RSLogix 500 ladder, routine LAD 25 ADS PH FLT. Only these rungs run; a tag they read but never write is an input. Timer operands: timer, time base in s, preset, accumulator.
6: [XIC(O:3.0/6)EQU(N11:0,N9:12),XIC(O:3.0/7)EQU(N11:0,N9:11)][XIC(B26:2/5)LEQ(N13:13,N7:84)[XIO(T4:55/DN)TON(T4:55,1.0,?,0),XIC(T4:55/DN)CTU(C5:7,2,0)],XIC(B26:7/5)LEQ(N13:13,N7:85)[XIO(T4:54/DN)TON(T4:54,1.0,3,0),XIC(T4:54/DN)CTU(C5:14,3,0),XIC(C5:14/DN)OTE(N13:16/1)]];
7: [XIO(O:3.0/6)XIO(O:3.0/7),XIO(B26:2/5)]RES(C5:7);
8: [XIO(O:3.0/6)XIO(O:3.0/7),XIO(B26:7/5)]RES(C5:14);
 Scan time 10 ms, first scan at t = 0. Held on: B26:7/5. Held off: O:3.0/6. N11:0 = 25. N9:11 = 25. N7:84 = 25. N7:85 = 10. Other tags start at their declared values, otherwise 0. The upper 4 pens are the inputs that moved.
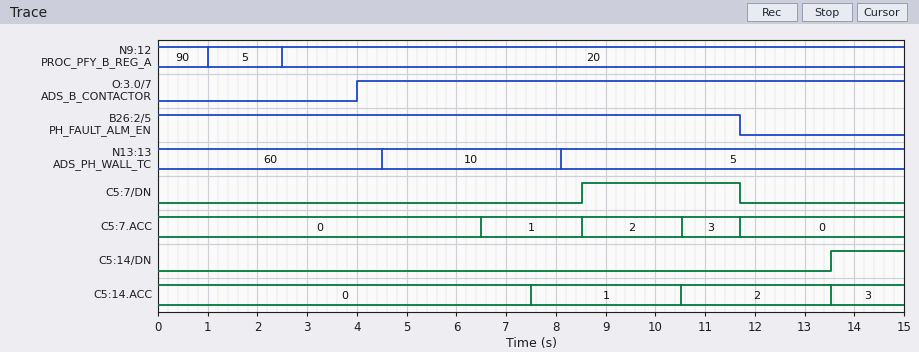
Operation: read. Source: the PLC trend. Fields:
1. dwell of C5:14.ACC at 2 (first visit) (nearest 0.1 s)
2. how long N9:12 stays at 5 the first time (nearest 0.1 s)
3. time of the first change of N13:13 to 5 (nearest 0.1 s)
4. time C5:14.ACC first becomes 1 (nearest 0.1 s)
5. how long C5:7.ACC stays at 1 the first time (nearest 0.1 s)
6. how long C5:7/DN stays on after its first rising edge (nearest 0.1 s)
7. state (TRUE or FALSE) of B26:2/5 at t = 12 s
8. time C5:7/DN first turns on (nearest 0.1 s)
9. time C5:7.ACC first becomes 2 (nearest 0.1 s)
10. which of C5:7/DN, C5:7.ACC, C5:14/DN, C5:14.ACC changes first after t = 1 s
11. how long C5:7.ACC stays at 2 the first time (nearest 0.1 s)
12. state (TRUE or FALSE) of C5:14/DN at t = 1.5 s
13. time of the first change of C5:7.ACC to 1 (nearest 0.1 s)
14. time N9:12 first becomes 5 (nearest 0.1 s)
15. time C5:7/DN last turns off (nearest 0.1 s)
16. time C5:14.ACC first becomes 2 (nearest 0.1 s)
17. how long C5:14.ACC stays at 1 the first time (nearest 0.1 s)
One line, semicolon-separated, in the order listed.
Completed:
3.0 s; 1.5 s; 8.1 s; 7.5 s; 2.0 s; 3.2 s; FALSE; 8.5 s; 8.5 s; C5:7.ACC; 2.0 s; FALSE; 6.5 s; 1.0 s; 11.7 s; 10.5 s; 3.0 s
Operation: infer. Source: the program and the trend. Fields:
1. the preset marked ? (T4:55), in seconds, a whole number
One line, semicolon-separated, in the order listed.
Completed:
2 s
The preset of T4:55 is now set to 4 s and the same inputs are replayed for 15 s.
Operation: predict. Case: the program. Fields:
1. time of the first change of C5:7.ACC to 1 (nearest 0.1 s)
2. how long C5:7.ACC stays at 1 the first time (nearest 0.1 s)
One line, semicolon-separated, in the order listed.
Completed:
8.5 s; 3.2 s
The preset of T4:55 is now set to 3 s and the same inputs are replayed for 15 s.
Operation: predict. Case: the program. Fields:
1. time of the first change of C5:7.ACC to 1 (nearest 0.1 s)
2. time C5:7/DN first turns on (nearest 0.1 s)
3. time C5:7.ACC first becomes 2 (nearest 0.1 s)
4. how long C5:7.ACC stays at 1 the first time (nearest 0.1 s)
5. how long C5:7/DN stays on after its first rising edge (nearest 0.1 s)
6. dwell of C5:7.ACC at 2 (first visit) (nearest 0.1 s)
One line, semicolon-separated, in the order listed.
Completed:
7.5 s; 10.5 s; 10.5 s; 3.0 s; 1.2 s; 1.2 s
